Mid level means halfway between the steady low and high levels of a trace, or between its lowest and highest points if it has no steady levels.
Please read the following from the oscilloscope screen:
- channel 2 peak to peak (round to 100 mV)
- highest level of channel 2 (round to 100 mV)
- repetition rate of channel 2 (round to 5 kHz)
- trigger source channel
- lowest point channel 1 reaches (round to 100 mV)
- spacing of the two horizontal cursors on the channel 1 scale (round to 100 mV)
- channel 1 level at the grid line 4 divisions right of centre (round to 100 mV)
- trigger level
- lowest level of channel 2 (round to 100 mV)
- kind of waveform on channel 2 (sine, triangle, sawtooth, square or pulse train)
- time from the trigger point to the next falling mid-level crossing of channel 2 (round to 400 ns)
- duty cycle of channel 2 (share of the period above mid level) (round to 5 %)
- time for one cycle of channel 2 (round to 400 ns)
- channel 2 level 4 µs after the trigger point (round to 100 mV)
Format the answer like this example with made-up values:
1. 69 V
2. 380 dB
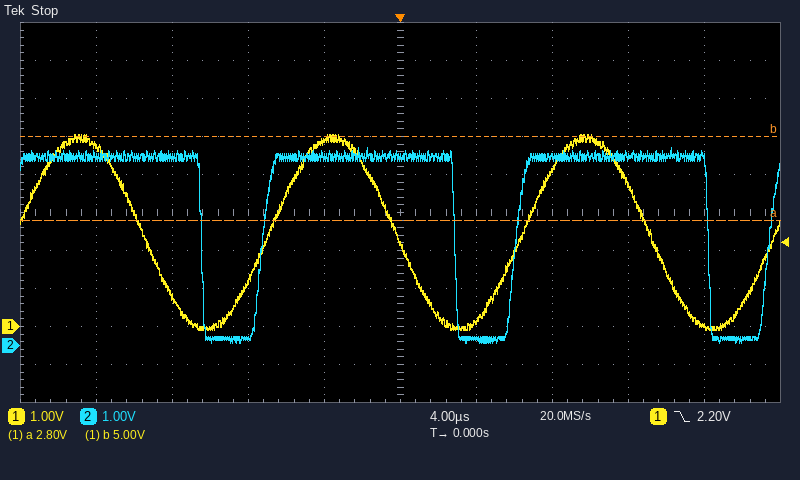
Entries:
1. 5.1 V
2. 5.2 V
3. 75 kHz
4. channel 1
5. -100 mV
6. 2.2 V
7. 0.0 V
8. 2.20 V
9. 100 mV
10. pulse train
11. 2.8 µs
12. 75 %
13. 13.2 µs
14. 200 mV
